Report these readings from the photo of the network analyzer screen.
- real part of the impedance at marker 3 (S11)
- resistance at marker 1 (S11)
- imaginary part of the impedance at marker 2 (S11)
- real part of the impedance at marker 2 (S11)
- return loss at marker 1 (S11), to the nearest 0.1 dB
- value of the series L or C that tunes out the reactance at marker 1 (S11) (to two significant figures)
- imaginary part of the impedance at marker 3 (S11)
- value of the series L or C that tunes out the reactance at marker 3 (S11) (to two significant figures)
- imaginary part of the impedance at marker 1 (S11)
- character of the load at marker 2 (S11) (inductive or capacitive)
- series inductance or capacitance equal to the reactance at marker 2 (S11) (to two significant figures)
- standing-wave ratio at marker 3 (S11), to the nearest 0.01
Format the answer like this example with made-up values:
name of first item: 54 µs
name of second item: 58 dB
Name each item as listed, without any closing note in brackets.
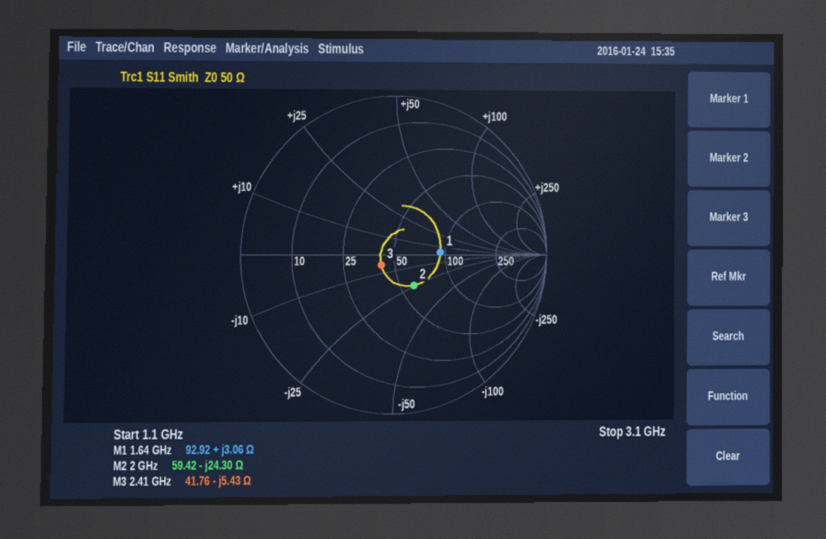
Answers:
real part of the impedance at marker 3: 41.76 Ω
resistance at marker 1: 92.92 Ω
imaginary part of the impedance at marker 2: -24.30 Ω
real part of the impedance at marker 2: 59.42 Ω
return loss at marker 1 (S11), to the nearest 0.1 dB: 10.4 dB
value of the series L or C that tunes out the reactance at marker 1 (S11): 32 pF
imaginary part of the impedance at marker 3: -5.43 Ω
value of the series L or C that tunes out the reactance at marker 3 (S11): 360 pH
imaginary part of the impedance at marker 1: +3.06 Ω
character of the load at marker 2 (S11): capacitive
series inductance or capacitance equal to the reactance at marker 2 (S11): 3.3 pF
standing-wave ratio at marker 3 (S11), to the nearest 0.01: 1.24
